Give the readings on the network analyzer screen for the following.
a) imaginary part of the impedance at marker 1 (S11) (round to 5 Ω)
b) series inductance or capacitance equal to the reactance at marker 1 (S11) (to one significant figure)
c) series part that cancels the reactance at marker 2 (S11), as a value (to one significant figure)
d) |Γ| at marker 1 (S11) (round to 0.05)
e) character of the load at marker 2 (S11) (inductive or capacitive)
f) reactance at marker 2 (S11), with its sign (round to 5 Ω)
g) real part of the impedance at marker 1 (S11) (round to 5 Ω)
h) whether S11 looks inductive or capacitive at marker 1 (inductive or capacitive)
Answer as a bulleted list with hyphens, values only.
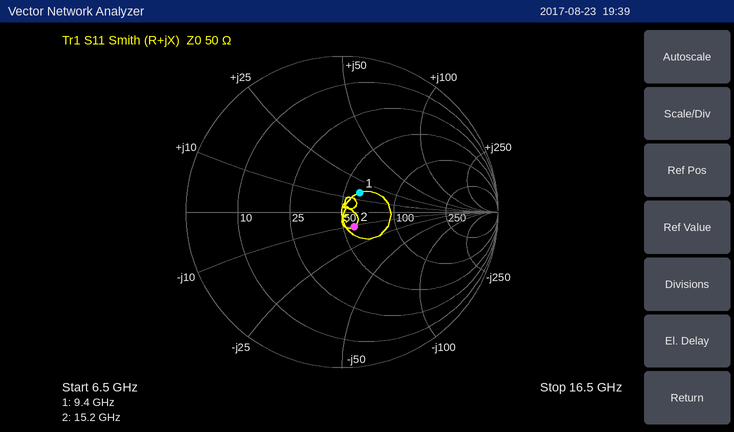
- +15 Ω
- 300 pH
- 100 pH
- 0.15
- capacitive
- -10 Ω
- 60 Ω
- inductive
